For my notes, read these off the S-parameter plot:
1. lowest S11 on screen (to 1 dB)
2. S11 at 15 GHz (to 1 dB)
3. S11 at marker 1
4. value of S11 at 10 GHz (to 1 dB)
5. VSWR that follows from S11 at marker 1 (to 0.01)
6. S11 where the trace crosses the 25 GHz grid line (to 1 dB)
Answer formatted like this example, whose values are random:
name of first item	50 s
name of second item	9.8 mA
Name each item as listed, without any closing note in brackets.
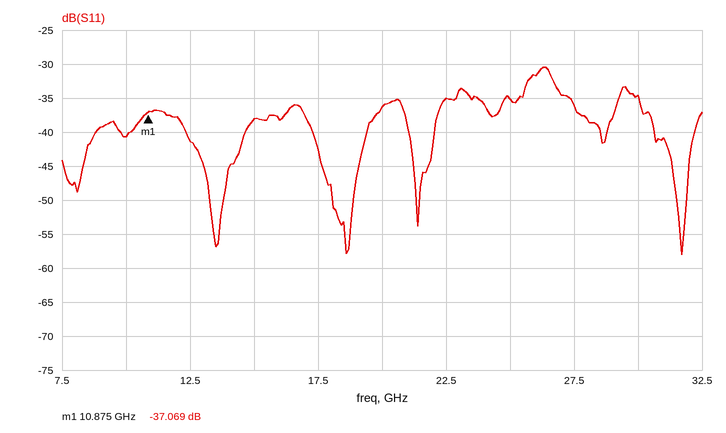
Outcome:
lowest S11 on screen	-58 dB
S11 at 15 GHz	-38 dB
S11 at marker 1	-37.069 dB
value of S11 at 10 GHz	-41 dB
VSWR that follows from S11 at marker 1	1.03
S11 where the trace crosses the 25 GHz grid line	-35 dB
